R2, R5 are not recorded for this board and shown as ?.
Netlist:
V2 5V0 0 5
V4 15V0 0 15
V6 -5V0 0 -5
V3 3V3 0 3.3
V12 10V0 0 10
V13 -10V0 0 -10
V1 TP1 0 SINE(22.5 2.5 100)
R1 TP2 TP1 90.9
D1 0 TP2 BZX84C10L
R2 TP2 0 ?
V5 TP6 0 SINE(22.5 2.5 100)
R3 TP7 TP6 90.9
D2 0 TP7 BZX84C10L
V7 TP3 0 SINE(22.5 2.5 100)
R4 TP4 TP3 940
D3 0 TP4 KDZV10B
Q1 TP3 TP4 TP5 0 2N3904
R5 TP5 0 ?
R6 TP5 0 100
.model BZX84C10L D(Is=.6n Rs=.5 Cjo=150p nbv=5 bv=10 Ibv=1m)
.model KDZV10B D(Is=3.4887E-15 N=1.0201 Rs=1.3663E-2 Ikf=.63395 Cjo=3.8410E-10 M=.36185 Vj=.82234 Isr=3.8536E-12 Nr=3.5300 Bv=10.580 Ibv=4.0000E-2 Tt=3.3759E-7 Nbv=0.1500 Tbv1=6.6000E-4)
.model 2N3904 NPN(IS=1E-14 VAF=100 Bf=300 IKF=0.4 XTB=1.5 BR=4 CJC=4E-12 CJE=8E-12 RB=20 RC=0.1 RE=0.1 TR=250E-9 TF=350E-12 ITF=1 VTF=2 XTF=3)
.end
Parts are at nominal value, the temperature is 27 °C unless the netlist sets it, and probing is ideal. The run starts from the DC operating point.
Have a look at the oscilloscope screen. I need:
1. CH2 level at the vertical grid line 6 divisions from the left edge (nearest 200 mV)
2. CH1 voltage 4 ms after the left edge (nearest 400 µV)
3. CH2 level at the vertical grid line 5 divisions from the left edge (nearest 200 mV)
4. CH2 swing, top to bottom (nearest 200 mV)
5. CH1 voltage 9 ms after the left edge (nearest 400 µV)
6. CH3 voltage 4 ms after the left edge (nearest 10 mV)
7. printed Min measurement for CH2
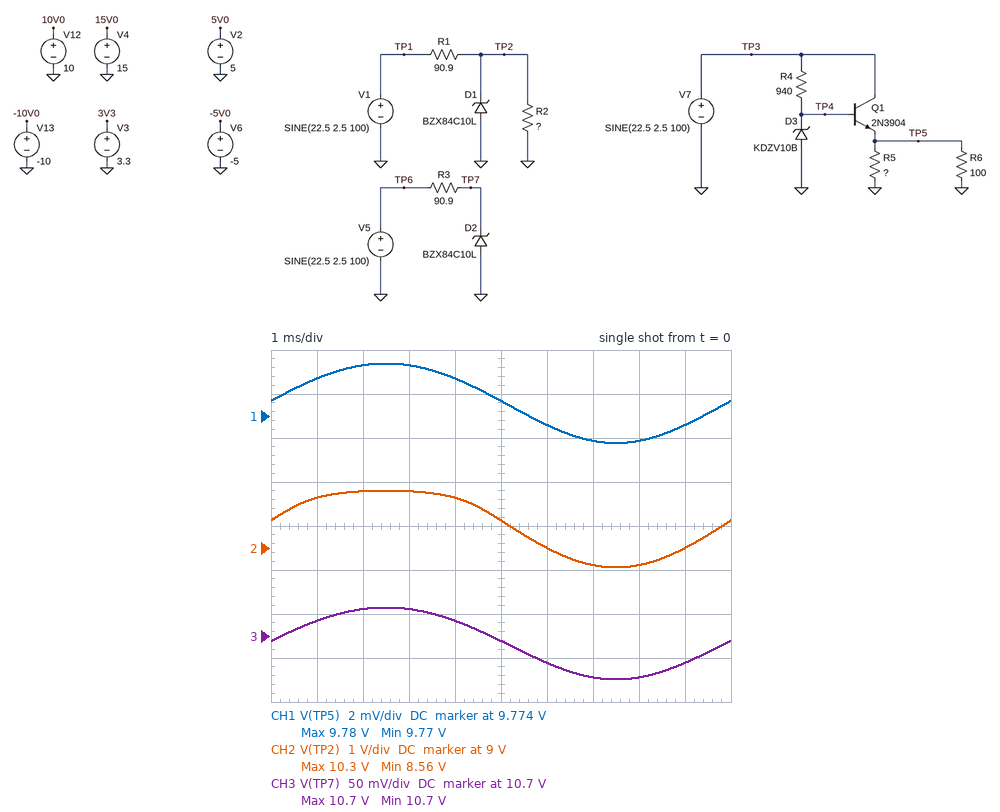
9.0 V
9.7756 V
9.6 V
1.8 V
9.7736 V
10.72 V
8.56 V
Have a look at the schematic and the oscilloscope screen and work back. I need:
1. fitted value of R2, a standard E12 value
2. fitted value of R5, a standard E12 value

68 Ω
560 Ω
